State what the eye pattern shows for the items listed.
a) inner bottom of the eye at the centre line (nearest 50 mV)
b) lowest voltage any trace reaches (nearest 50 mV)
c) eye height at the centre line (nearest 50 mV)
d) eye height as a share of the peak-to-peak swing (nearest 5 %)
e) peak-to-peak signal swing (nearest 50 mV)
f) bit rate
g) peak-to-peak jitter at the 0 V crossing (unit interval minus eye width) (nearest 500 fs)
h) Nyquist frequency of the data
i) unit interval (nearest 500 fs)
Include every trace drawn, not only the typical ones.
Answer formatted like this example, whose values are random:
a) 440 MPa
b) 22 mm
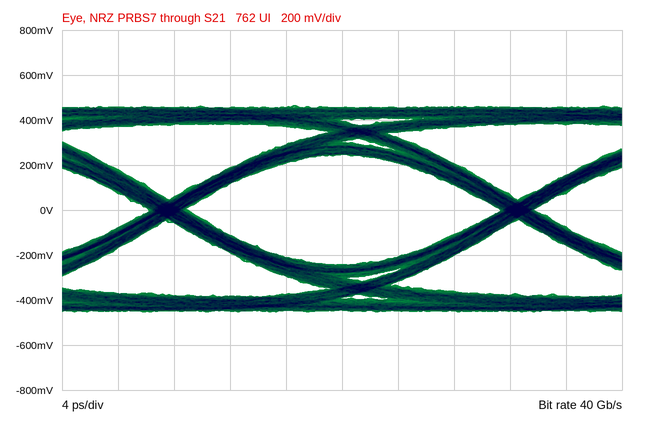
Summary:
a) -250 mV
b) -450 mV
c) 500 mV
d) 55 %
e) 900 mV
f) 40 Gb/s
g) 2.5 ps
h) 20 GHz
i) 25.0 ps
